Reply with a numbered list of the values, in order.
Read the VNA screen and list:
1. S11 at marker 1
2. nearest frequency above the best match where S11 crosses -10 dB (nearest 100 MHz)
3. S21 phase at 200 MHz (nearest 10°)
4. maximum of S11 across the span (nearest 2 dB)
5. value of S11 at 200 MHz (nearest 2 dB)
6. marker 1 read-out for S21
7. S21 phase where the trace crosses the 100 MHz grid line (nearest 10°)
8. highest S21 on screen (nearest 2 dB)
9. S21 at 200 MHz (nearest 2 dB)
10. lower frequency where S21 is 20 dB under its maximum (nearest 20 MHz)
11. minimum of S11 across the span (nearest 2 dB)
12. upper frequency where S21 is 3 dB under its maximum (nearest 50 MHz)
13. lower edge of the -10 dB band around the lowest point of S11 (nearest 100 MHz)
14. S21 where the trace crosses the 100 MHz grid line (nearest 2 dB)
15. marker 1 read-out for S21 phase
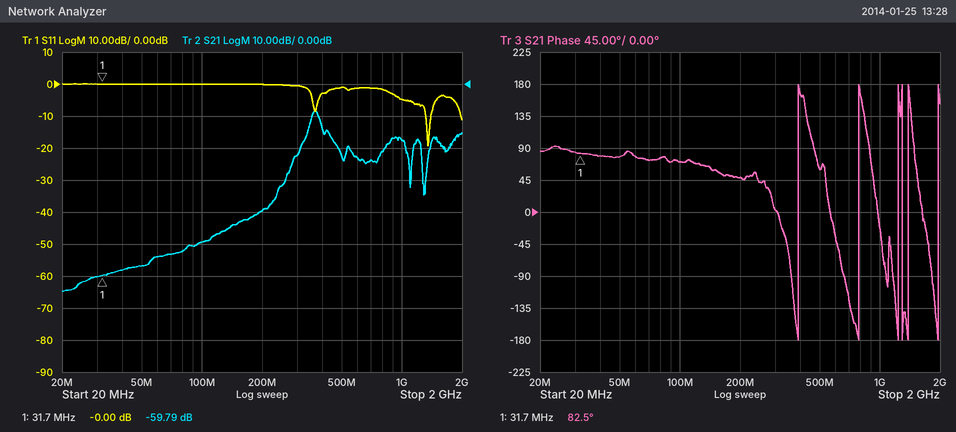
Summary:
1. -0.00 dB
2. 1.4 GHz
3. 50°
4. 0 dB
5. 0 dB
6. -59.79 dB
7. 70°
8. -8 dB
9. -40 dB
10. 260 MHz
11. -20 dB
12. 400 MHz
13. 1.3 GHz
14. -50 dB
15. 82.5°
